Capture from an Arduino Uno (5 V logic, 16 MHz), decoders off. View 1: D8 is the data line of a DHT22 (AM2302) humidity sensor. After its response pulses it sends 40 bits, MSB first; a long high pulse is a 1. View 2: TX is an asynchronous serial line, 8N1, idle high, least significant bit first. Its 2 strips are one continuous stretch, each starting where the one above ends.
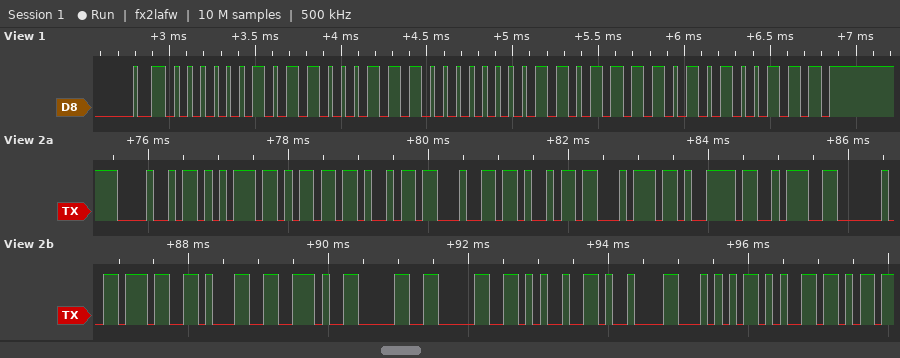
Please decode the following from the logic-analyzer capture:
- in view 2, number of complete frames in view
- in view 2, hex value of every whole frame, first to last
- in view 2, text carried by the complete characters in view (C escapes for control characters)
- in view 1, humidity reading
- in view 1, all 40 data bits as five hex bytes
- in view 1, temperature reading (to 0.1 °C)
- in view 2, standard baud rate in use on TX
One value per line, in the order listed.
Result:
19
0x48 0x75 0x6D 0x69 0x64 0x69 0x74 0x79 0x3A 0x20 0x37 0x31 0x2E 0x30 0x30 0x25 0x09 0x54 0x65
"Humidity: 71.00%\tTe"
71.1 %
02 C7 00 DE A7
22.2 °C
9600 baud
